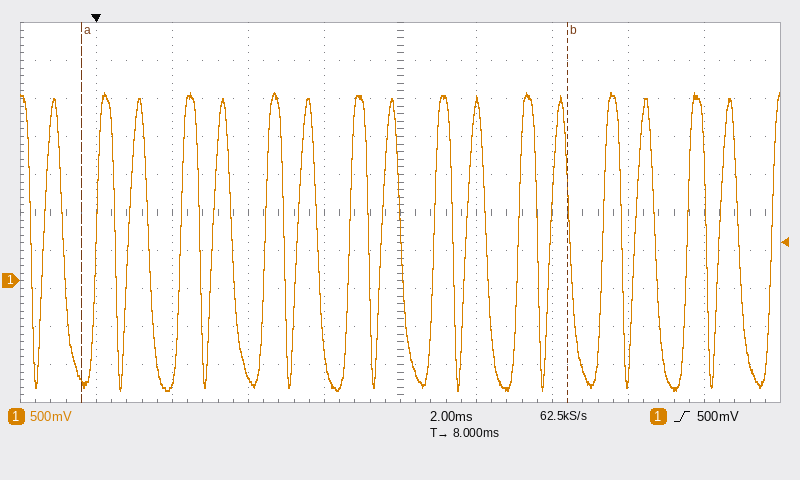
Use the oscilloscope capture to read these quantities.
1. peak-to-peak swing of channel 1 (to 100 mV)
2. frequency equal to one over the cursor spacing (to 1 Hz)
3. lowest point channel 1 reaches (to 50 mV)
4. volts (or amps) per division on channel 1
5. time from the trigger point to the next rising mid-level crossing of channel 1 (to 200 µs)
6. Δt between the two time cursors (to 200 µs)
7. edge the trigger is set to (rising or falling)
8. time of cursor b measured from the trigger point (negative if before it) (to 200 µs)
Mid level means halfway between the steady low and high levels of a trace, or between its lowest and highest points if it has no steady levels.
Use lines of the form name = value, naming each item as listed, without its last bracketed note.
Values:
peak-to-peak swing of channel 1 = 3.90 V
frequency equal to one over the cursor spacing = 78 Hz
lowest point channel 1 reaches = -1.45 V
volts (or amps) per division on channel 1 = 500 mV
time from the trigger point to the next rising mid-level crossing of channel 1 = 800 µs
Δt between the two time cursors = 12.8 ms
edge the trigger is set to = rising
time of cursor b measured from the trigger point (negative if before it) = +12.4 ms
